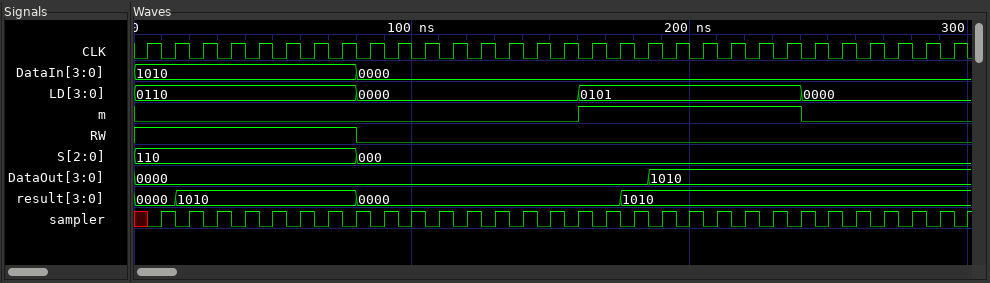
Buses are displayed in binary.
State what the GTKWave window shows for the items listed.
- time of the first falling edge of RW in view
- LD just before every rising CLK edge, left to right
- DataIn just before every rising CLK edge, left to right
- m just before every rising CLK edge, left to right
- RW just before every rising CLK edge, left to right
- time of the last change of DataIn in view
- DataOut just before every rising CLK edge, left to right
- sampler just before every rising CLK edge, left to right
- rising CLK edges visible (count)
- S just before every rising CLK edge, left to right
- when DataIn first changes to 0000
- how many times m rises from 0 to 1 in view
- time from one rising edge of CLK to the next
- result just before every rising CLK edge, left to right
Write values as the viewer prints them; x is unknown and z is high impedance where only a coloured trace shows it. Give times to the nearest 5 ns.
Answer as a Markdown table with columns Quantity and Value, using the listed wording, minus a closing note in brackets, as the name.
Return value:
| Quantity | Value |
|---|---|
| time of the first falling edge of RW in view | 80 ns |
| LD just before every rising CLK edge, left to right | 0110, 0110, 0110, 0110, 0110, 0110, 0110, 0110, 0000, 0000, 0000, 0000, 0000, 0000, 0000, 0000, 0101, 0101, 0101, 0101, 0101, 0101, 0101, 0101, 0000, 0000, 0000, 0000, 0000, 0000 |
| DataIn just before every rising CLK edge, left to right | 1010, 1010, 1010, 1010, 1010, 1010, 1010, 1010, 0000, 0000, 0000, 0000, 0000, 0000, 0000, 0000, 0000, 0000, 0000, 0000, 0000, 0000, 0000, 0000, 0000, 0000, 0000, 0000, 0000, 0000 |
| m just before every rising CLK edge, left to right | 0 0 0 0 0 0 0 0 0 0 0 0 0 0 0 0 1 1 1 1 1 1 1 1 0 0 0 0 0 0 |
| RW just before every rising CLK edge, left to right | 1 1 1 1 1 1 1 1 0 0 0 0 0 0 0 0 0 0 0 0 0 0 0 0 0 0 0 0 0 0 |
| time of the last change of DataIn in view | 80 ns |
| DataOut just before every rising CLK edge, left to right | 0000, 0000, 0000, 0000, 0000, 0000, 0000, 0000, 0000, 0000, 0000, 0000, 0000, 0000, 0000, 0000, 0000, 0000, 0000, 1010, 1010, 1010, 1010, 1010, 1010, 1010, 1010, 1010, 1010, 1010 |
| sampler just before every rising CLK edge, left to right | x 1 1 1 1 1 1 1 1 1 1 1 1 1 1 1 1 1 1 1 1 1 1 1 1 1 1 1 1 1 |
| rising CLK edges visible | 30 |
| S just before every rising CLK edge, left to right | 110, 110, 110, 110, 110, 110, 110, 110, 000, 000, 000, 000, 000, 000, 000, 000, 000, 000, 000, 000, 000, 000, 000, 000, 000, 000, 000, 000, 000, 000 |
| when DataIn first changes to 0000 | 80 ns |
| how many times m rises from 0 to 1 in view | 1 |
| time from one rising edge of CLK to the next | 10 ns |
| result just before every rising CLK edge, left to right | 0000, 0000, 1010, 1010, 1010, 1010, 1010, 1010, 0000, 0000, 0000, 0000, 0000, 0000, 0000, 0000, 0000, 0000, 1010, 1010, 1010, 1010, 1010, 1010, 1010, 1010, 1010, 1010, 1010, 1010 |
